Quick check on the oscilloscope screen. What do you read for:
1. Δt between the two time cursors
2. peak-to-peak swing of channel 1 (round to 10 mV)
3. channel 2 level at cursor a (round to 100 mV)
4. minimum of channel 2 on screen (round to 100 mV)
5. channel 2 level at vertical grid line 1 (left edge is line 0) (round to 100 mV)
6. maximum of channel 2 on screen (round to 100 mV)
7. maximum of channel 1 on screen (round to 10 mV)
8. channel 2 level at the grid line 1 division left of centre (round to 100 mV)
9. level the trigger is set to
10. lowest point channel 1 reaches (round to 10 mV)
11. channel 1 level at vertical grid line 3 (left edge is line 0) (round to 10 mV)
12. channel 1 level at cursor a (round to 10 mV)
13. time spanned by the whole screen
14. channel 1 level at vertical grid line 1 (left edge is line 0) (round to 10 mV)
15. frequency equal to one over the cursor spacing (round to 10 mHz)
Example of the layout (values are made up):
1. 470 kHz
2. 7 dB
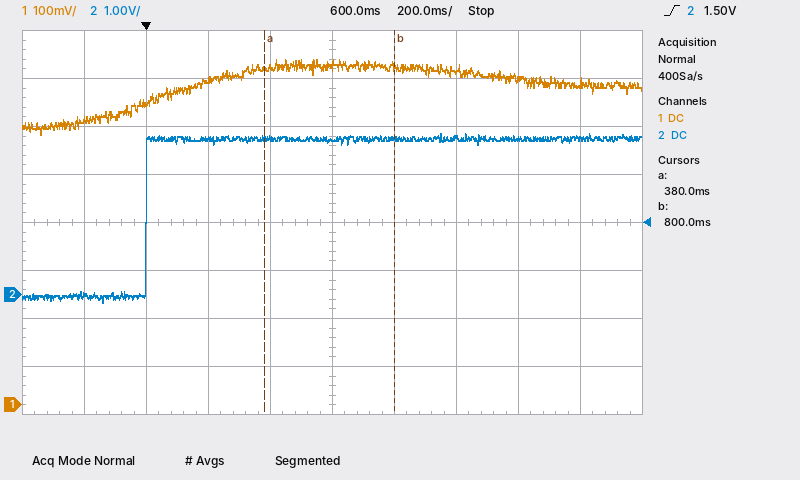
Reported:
1. 420 ms
2. 160 mV
3. 3.3 V
4. -200 mV
5. 0.0 V
6. 3.4 V
7. 720 mV
8. 3.3 V
9. 1.50 V
10. 560 mV
11. 680 mV
12. 700 mV
13. 2 s
14. 590 mV
15. 2.38 Hz
